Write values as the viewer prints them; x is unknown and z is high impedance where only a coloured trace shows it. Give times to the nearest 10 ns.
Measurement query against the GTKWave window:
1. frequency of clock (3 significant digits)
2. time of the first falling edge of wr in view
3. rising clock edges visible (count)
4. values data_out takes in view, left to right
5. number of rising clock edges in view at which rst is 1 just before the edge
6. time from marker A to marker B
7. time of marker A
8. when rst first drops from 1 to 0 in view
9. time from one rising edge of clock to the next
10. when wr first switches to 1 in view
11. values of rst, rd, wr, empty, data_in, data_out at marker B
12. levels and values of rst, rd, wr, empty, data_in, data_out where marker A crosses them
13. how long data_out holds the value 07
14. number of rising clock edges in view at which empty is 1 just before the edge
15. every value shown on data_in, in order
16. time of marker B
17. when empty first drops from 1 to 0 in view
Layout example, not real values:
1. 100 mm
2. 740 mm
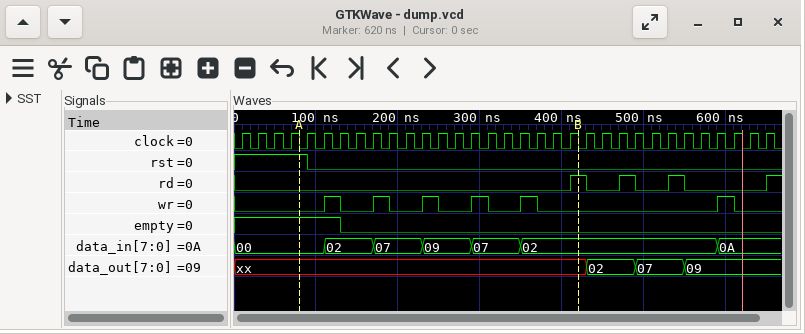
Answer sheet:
1. 50.0 MHz
2. 130 ns
3. 33
4. xx, 02, 07, 09
5. 5
6. 340 ns
7. 80 ns
8. 90 ns
9. 20 ns
10. 110 ns
11. rst=0, rd=1, wr=0, empty=0, data_in=02, data_out=xx
12. rst=1, rd=0, wr=0, empty=1, data_in=00, data_out=xx
13. 60 ns
14. 7
15. 00, 02, 07, 09, 07, 02, 0A
16. 420 ns
17. 130 ns
